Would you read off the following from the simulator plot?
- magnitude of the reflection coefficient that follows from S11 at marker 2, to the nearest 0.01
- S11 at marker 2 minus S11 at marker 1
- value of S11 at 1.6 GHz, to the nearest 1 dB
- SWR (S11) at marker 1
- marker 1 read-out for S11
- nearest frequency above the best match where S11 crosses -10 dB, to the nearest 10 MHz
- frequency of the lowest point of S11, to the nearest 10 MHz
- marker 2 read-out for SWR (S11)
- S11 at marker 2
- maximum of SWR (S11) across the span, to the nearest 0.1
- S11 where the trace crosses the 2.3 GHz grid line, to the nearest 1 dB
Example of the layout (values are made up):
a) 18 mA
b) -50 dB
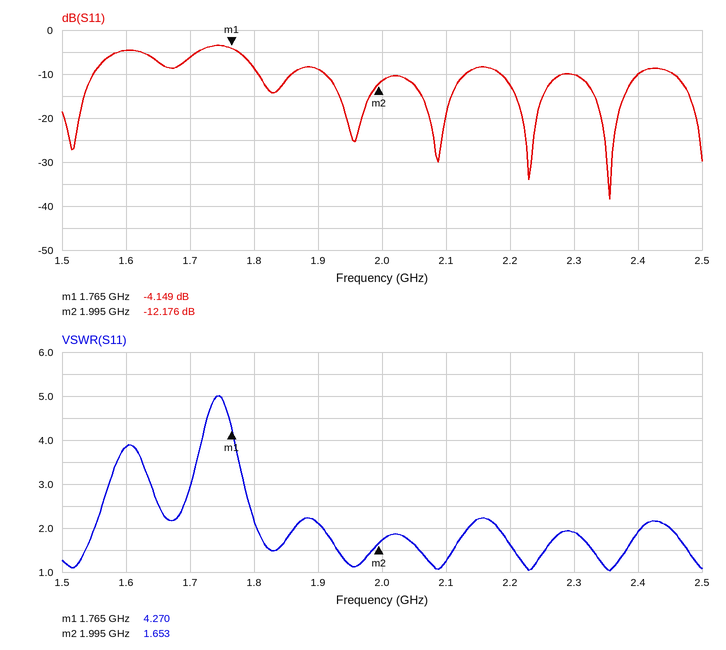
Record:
a) 0.25
b) -8.027 dB
c) -5 dB
d) 4.270
e) -4.149 dB
f) 2.40 GHz
g) 2.36 GHz
h) 1.653
i) -12.176 dB
j) 5.0
k) -10 dB
